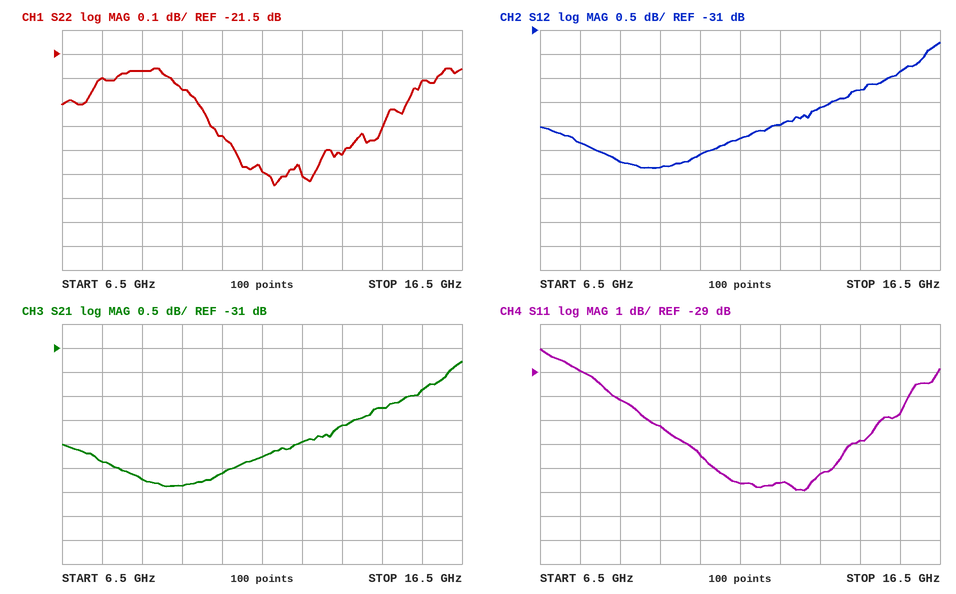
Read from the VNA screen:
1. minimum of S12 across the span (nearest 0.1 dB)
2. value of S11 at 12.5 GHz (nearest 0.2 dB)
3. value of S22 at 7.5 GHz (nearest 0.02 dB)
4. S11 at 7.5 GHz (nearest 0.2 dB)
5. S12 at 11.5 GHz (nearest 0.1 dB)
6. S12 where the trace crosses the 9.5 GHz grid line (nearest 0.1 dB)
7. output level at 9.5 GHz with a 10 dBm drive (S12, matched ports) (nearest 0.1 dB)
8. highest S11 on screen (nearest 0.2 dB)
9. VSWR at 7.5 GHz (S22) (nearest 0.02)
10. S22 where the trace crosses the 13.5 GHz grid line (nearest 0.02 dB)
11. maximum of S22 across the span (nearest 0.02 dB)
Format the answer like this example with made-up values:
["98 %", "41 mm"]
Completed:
["-33.9 dB", "-33.6 dB", "-21.60 dB", "-29.0 dB", "-33.3 dB", "-33.9 dB", "-23.9 dBm", "-28.0 dB", "1.18", "-21.92 dB", "-21.56 dB"]
